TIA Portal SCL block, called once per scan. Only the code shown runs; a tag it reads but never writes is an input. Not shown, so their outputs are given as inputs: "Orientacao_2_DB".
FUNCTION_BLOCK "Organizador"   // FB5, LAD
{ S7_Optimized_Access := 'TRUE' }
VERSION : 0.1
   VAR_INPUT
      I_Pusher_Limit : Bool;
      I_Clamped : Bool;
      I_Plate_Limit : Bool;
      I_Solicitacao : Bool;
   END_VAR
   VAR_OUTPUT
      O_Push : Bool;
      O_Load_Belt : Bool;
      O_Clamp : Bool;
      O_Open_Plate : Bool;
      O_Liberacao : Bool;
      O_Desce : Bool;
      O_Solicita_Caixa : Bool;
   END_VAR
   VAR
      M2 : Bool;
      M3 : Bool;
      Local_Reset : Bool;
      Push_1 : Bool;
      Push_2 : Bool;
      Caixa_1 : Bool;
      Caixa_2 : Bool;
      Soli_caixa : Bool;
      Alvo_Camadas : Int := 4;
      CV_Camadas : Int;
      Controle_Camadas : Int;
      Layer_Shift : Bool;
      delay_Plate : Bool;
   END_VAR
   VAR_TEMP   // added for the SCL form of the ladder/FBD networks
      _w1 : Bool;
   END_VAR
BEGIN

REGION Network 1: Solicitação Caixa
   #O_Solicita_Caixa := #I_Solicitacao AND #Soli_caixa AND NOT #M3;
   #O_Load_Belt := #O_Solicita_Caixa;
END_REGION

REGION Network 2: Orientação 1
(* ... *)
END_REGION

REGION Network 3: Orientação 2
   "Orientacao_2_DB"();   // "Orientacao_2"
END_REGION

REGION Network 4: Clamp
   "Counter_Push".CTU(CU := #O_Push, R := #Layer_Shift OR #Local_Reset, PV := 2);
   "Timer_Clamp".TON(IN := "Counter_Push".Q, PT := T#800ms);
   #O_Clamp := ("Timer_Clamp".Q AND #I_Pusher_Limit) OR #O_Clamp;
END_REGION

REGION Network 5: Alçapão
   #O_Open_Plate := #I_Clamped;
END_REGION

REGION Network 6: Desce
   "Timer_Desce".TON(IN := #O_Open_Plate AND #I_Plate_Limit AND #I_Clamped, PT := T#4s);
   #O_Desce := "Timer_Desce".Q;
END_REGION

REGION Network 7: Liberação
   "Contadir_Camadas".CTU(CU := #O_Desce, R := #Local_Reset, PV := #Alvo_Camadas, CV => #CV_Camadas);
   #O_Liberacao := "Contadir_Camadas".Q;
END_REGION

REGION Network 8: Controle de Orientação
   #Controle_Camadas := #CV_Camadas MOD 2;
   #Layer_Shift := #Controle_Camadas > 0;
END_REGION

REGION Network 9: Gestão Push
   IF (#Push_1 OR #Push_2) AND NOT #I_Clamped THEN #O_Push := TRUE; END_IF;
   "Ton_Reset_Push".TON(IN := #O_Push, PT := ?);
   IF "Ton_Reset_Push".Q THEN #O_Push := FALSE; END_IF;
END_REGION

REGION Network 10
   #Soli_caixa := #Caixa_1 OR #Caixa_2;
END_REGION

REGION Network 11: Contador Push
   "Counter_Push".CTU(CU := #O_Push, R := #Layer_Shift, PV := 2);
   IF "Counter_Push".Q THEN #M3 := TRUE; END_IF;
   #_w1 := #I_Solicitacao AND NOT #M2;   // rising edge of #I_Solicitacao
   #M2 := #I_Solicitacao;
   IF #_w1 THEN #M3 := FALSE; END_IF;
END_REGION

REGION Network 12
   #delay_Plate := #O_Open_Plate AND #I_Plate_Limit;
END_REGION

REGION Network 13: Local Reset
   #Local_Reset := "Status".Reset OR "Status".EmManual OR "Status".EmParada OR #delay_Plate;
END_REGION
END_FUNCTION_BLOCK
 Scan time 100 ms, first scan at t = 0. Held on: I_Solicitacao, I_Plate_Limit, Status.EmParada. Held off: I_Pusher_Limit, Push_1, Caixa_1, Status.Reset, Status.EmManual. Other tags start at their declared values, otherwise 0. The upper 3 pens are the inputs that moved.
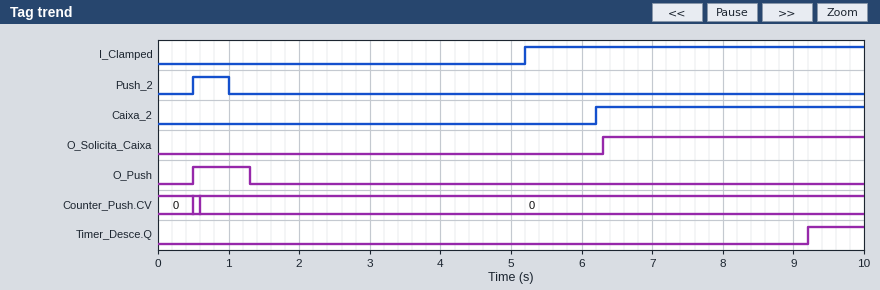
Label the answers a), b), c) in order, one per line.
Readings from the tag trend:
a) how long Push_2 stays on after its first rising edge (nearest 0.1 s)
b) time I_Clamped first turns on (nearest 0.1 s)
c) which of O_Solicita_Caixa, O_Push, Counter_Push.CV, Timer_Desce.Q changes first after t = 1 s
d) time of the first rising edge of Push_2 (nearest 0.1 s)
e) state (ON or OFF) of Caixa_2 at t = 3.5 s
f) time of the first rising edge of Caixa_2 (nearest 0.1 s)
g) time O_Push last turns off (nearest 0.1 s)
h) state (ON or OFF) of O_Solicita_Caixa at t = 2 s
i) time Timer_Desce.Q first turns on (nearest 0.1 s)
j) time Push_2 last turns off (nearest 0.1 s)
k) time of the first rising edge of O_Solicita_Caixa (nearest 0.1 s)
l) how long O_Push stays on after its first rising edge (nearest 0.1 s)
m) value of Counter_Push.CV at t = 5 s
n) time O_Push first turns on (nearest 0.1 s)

a) 0.5 s
b) 5.2 s
c) O_Push
d) 0.5 s
e) OFF
f) 6.2 s
g) 1.3 s
h) OFF
i) 9.2 s
j) 1.0 s
k) 6.3 s
l) 0.8 s
m) 0
n) 0.5 s
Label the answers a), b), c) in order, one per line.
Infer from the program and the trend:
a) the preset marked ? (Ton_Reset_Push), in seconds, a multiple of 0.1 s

a) 0.8 s
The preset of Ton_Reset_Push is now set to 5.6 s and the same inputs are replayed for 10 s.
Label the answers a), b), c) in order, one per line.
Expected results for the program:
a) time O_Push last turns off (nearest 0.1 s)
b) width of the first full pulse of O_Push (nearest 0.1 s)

a) 6.1 s
b) 5.6 s
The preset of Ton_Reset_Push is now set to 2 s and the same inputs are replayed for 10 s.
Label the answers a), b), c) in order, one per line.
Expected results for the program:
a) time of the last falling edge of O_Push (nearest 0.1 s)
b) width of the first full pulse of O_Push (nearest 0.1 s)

a) 2.5 s
b) 2.0 s
